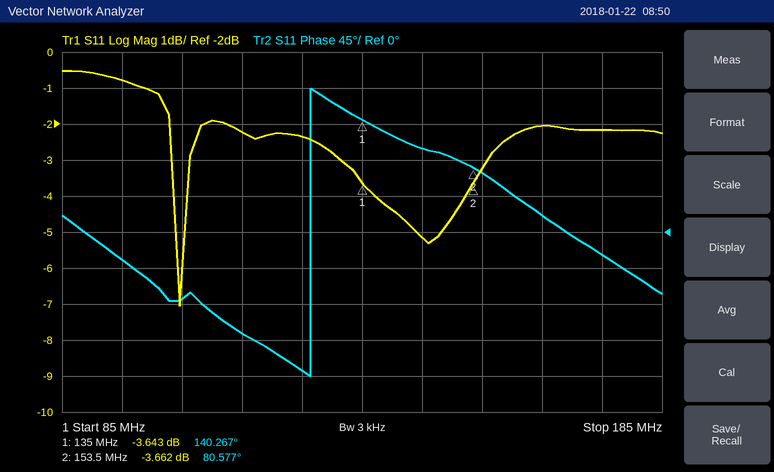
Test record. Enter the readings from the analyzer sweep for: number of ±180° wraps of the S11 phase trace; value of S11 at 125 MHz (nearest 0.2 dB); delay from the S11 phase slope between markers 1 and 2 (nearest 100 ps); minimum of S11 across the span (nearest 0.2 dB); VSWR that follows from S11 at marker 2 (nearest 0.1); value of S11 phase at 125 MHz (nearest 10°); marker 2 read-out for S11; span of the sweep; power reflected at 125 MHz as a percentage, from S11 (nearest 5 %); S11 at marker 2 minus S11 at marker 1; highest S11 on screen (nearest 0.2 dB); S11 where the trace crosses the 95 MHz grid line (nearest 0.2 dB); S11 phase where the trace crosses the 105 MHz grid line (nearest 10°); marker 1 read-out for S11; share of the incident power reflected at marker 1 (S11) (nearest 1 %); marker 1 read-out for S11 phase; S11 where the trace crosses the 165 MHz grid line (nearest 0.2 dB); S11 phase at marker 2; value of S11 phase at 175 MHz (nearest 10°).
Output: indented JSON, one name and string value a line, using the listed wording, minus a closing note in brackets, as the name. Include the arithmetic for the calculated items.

{
  "number of ±180° wraps of the S11 phase trace": "1",
  "value of S11 at 125 MHz": "-2.4 dB",
  "delay from the S11 phase slope between markers 1 and 2": "−(80.577° − (140.267°))/(360° × 18.5 MHz) ≈ 9.0 ns",
  "minimum of S11 across the span": "-7.0 dB",
  "VSWR that follows from S11 at marker 2": "(1 + 0.6560)/(1 − 0.6560) ≈ 4.8",
  "value of S11 phase at 125 MHz": "-170°",
  "marker 2 read-out for S11": "-3.662 dB",
  "span of the sweep": "100 MHz",
  "power reflected at 125 MHz as a percentage, from S11": "10^(-2.4/10) ≈ 57.5 %, so 60 % to the nearest 5 %",
  "S11 at marker 2 minus S11 at marker 1": "-3.662 − (-3.643) = -0.019 dB",
  "highest S11 on screen": "-0.6 dB",
  "S11 where the trace crosses the 95 MHz grid line": "-0.8 dB",
  "S11 phase where the trace crosses the 105 MHz grid line": "-80°",
  "marker 1 read-out for S11": "-3.643 dB",
  "share of the incident power reflected at marker 1 (S11)": "10^(-3.643/10) ≈ 43 %",
  "marker 1 read-out for S11 phase": "140.267°",
  "S11 where the trace crosses the 165 MHz grid line": "-2.0 dB",
  "S11 phase at marker 2": "80.577°",
  "value of S11 phase at 175 MHz": "-30°"
}
